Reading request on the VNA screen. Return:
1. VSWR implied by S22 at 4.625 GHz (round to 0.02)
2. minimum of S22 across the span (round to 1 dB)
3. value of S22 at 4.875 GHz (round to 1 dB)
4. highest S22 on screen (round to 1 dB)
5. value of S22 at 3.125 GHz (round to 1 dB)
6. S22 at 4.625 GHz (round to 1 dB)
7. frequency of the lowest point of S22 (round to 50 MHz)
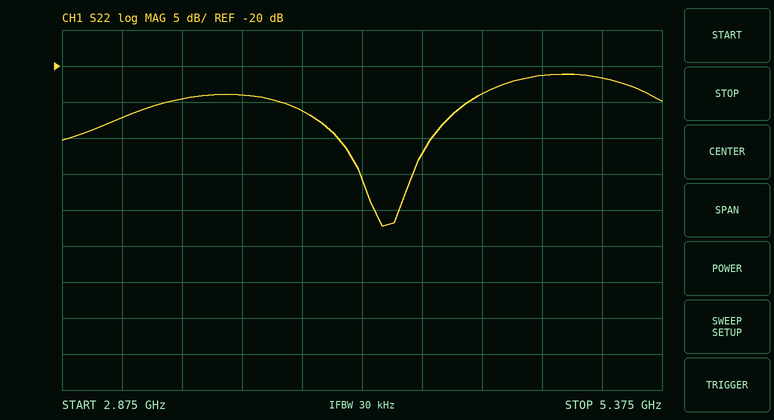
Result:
1.14
-42 dB
-21 dB
-21 dB
-27 dB
-24 dB
4.20 GHz
